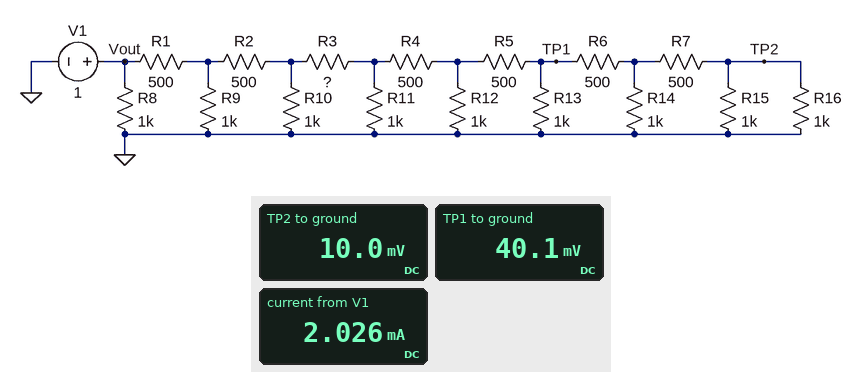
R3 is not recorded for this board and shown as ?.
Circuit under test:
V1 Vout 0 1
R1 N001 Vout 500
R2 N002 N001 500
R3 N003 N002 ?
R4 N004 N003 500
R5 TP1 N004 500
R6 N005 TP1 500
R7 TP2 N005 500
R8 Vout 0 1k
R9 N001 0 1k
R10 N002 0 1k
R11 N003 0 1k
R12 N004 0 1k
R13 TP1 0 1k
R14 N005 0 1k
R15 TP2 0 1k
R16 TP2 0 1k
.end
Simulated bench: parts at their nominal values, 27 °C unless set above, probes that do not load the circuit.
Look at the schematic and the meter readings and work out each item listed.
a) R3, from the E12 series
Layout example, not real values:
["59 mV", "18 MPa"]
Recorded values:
["180 Ω"]
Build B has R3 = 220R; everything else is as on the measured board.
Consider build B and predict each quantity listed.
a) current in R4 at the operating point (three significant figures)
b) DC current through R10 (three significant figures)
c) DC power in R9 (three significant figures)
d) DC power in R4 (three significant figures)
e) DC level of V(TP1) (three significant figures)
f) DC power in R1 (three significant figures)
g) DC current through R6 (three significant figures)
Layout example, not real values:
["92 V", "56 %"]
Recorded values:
["155 µA", "223 µA", "239 µW", "12.0 µW", "38.7 mV", "522 µW", "38.7 µA"]
